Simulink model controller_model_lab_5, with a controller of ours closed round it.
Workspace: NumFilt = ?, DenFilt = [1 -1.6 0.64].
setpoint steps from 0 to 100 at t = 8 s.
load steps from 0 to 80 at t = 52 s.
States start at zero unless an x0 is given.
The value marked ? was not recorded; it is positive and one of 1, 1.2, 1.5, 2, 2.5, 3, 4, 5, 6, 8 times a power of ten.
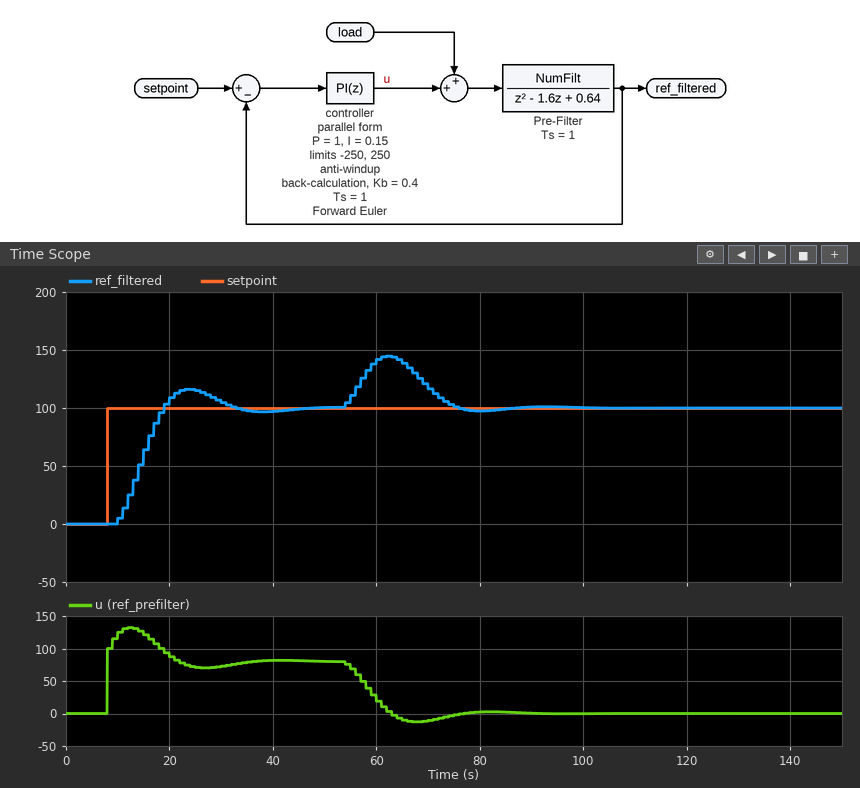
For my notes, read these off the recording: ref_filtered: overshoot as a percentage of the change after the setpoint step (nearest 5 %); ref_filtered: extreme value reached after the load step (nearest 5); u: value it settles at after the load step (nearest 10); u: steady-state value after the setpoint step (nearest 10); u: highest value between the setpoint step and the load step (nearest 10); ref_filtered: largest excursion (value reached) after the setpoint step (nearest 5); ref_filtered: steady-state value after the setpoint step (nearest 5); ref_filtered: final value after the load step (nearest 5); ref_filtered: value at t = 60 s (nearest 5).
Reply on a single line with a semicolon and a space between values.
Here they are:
15 %; 145; 0; 80; 130; 115; 100; 100; 140
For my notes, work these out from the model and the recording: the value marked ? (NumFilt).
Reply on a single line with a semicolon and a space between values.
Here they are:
0.05
